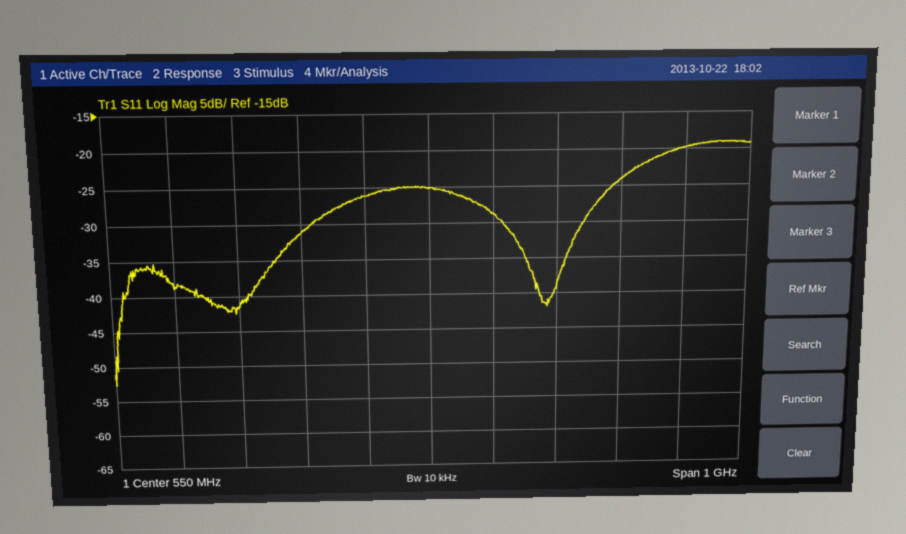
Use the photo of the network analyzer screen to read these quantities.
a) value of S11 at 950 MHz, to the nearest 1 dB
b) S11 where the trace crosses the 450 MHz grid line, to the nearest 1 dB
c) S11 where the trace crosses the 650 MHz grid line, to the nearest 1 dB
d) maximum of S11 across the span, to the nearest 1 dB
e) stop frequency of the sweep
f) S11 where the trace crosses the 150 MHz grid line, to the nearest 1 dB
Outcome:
-20 dB
-26 dB
-29 dB
-19 dB
1.05 GHz
-39 dB
